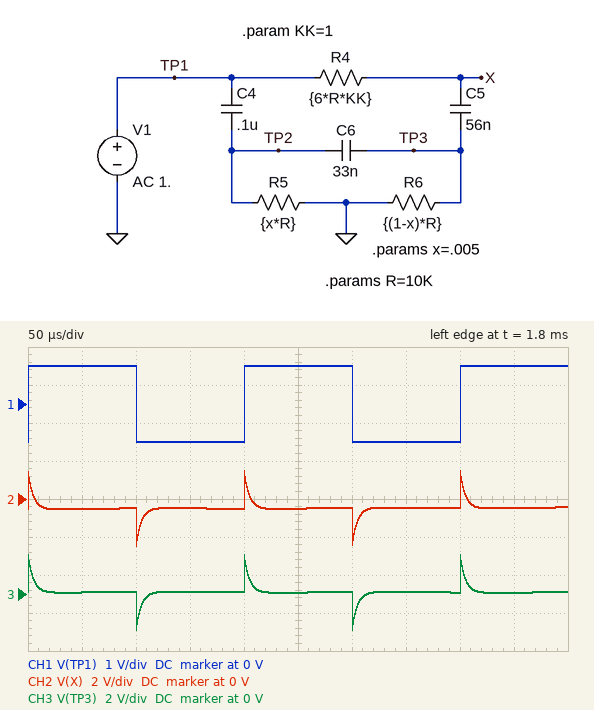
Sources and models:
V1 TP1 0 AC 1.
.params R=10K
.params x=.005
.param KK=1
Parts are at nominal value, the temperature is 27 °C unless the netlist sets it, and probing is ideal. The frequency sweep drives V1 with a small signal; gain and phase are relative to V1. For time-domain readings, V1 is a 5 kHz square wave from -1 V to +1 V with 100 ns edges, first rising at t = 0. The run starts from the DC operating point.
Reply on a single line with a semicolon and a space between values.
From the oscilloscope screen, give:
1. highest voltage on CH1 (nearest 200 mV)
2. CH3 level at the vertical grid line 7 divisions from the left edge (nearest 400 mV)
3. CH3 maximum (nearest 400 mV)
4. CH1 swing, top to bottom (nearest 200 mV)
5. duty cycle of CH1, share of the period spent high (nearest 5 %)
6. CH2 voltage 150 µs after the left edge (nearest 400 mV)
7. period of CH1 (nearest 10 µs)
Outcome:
1.0 V; 0 V; 2.0 V; 2.0 V; 50 %; -400 mV; 200 µs
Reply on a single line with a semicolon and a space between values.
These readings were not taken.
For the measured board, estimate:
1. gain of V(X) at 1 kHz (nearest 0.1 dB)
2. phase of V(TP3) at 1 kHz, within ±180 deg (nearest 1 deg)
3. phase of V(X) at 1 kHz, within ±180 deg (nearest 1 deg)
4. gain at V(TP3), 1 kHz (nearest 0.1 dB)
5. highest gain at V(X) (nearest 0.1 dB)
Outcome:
-21.4 dB; -54 deg; -70 deg; -27.4 dB; 0 dB
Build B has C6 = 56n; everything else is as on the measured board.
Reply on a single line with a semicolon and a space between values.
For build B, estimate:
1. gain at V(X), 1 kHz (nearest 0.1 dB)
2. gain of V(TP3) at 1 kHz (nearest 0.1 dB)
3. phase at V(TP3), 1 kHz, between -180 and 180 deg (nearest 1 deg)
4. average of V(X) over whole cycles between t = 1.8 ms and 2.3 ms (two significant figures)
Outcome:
-24.3 dB; -36.2 dB; -57 deg; -470 mV
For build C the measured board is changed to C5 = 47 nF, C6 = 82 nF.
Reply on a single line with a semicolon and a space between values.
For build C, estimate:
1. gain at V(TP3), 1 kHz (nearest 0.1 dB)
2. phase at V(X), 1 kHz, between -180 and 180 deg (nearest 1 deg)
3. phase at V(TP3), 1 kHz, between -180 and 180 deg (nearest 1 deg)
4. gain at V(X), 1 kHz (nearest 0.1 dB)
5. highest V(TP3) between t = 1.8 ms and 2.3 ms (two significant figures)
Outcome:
-48.8 dB; -83 deg; 0 deg; -25.0 dB; 2.1 V
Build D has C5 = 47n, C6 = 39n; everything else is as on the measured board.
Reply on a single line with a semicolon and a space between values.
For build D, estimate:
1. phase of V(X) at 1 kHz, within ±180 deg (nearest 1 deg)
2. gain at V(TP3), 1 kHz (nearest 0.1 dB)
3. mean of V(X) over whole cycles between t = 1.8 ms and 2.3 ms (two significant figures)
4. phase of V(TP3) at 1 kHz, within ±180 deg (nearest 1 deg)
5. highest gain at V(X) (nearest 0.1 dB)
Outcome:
-74 deg; -29.6 dB; -450 mV; -56 deg; 0 dB
